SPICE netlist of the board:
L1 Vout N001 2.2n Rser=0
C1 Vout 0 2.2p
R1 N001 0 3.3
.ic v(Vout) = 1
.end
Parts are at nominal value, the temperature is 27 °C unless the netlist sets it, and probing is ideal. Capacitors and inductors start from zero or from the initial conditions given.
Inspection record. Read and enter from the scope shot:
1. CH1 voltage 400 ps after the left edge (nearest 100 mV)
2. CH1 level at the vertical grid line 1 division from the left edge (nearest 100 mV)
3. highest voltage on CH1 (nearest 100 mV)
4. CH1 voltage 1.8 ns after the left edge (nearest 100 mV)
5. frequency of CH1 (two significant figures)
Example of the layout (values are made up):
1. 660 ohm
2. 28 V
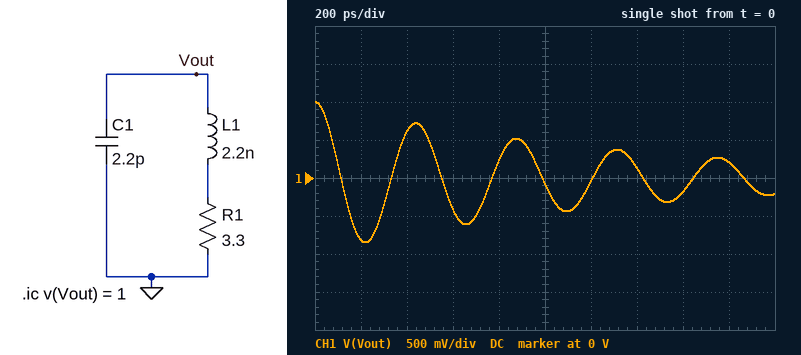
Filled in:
1. 600 mV
2. -800 mV
3. 1.0 V
4. 200 mV
5. 2.3 GHz
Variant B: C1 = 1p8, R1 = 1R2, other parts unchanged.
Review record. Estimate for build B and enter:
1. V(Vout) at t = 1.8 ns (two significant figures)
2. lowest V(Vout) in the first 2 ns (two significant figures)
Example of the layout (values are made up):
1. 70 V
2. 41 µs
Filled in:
1. -580 mV
2. -950 mV
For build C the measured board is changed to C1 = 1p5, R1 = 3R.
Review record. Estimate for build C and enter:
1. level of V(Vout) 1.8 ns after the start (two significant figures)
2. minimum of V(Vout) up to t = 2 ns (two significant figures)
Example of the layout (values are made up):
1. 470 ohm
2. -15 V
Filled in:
1. 290 mV
2. -880 mV
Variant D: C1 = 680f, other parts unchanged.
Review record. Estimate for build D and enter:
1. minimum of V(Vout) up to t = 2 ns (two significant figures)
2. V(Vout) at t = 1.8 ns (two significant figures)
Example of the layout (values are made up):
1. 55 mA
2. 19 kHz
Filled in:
1. -910 mV
2. -210 mV
